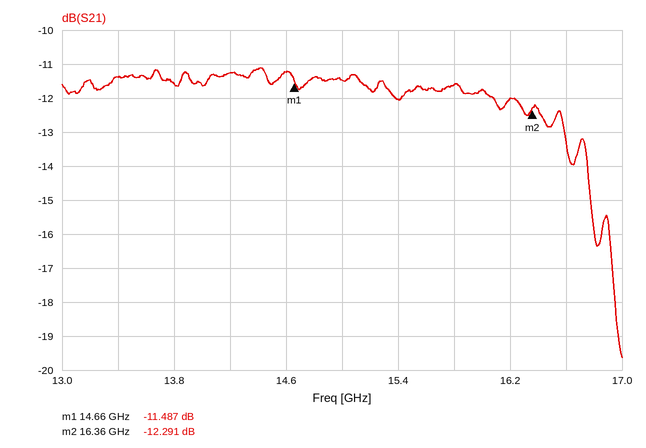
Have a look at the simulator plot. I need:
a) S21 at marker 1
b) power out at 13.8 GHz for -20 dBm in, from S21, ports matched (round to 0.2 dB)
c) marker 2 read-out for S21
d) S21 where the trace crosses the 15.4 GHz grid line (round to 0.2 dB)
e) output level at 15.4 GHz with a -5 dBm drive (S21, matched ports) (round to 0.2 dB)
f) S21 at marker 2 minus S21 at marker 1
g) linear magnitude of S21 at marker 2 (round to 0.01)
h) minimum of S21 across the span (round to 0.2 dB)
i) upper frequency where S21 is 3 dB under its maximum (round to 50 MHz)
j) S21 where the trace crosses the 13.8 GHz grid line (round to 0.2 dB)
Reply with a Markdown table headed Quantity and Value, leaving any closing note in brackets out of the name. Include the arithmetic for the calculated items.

| Quantity | Value |
|---|---|
| S21 at marker 1 | -11.487 dB |
| power out at 13.8 GHz for -20 dBm in, from S21, ports matched | -20 dBm + (-11.6 dB) = -31.6 dBm |
| marker 2 read-out for S21 | -12.291 dB |
| S21 where the trace crosses the 15.4 GHz grid line | -12.0 dB |
| output level at 15.4 GHz with a -5 dBm drive (S21, matched ports) | -5 dBm + (-12.0 dB) = -17.0 dBm |
| S21 at marker 2 minus S21 at marker 1 | -12.291 − (-11.487) = -0.804 dB |
| linear magnitude of S21 at marker 2 | 10^(-12.291/20) ≈ 0.24 |
| minimum of S21 across the span | -19.6 dB |
| upper frequency where S21 is 3 dB under its maximum | 16.75 GHz |
| S21 where the trace crosses the 13.8 GHz grid line | -11.6 dB |
